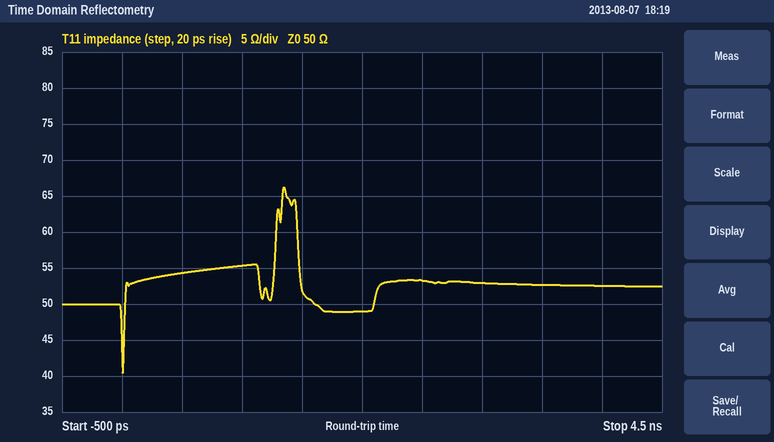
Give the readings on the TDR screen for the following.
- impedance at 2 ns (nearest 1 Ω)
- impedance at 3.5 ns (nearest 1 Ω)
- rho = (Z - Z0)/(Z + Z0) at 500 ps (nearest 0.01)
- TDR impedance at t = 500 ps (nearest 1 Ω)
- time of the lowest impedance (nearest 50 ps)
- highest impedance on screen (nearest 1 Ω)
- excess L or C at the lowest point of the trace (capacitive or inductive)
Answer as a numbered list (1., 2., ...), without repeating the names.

1. 49 Ω
2. 53 Ω
3. +0.04
4. 54 Ω
5. 0 ps
6. 66 Ω
7. capacitive
